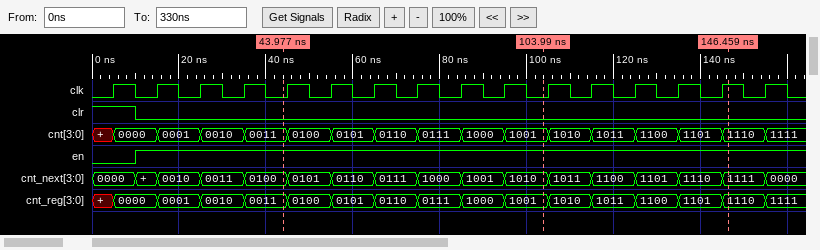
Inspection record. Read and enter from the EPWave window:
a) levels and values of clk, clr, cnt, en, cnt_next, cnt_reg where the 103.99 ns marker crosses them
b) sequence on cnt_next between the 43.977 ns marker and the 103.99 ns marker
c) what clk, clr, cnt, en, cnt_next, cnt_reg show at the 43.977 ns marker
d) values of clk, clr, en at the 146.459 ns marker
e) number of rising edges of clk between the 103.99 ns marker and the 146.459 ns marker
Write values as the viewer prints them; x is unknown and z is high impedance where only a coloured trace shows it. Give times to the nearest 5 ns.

clk=0, clr=0, cnt=1001, en=1, cnt_next=1010, cnt_reg=1001
0100, 0101, 0110, 0111, 1000, 1001, 1010
clk=0, clr=0, cnt=0011, en=1, cnt_next=0100, cnt_reg=0011
clk=1, clr=0, en=1
5
